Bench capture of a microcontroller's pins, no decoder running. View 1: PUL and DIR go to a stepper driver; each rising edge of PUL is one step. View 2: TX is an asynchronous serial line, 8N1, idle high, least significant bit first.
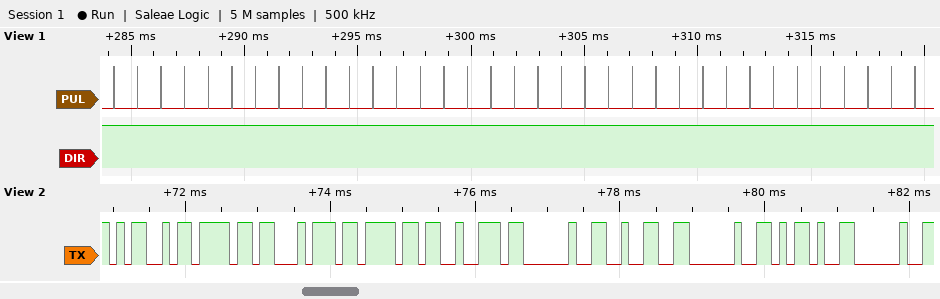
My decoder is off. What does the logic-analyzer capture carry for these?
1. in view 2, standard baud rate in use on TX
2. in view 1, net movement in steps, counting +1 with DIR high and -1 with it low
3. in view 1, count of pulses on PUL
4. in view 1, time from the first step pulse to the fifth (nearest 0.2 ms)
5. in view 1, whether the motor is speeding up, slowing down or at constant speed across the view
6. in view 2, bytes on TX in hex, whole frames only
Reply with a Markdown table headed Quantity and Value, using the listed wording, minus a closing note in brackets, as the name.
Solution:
| Quantity | Value |
|---|---|
| in view 2, standard baud rate in use on TX | 9600 baud |
| in view 1, net movement in steps, counting +1 with DIR high and -1 with it low | +35 |
| in view 1, count of pulses on PUL | 35 |
| in view 1, time from the first step pulse to the fifth | 4.2 ms |
| in view 1, whether the motor is speeding up, slowing down or at constant speed across the view | constant speed |
| in view 2, bytes on TX in hex, whole frames only | 0x4D 0x6F 0x74 0x6F 0x72 0x20 0x32 0x20 0x2D 0x20 |
